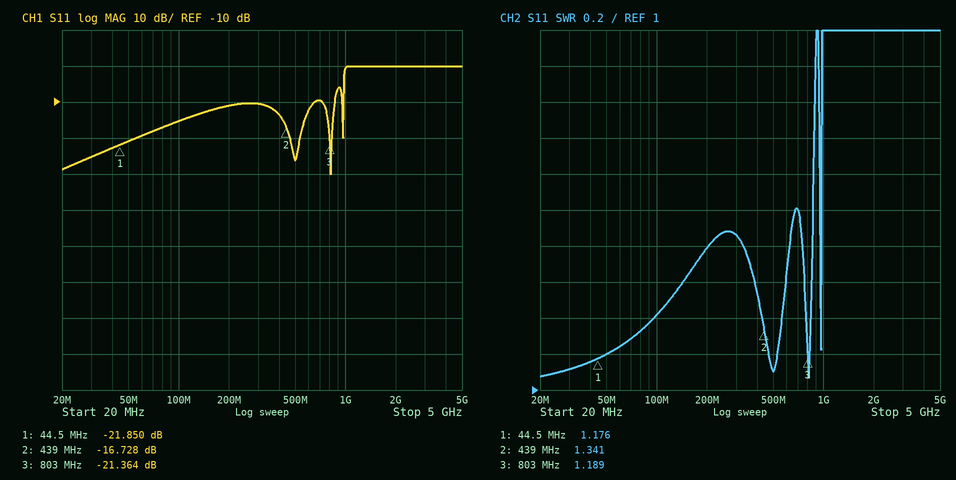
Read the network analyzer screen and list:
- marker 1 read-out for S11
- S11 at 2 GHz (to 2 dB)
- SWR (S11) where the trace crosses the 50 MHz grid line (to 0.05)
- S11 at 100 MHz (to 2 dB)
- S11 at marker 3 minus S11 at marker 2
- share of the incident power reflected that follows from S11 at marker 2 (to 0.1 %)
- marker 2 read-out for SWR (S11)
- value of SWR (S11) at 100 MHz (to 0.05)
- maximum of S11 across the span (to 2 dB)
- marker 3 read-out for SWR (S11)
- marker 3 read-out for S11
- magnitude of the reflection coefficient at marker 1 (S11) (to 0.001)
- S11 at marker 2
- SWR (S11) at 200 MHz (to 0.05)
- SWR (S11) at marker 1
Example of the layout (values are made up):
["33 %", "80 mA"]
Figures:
["-21.850 dB", "0 dB", "1.20", "-16 dB", "-4.636 dB", "2.1 %", "1.341", "1.40", "0 dB", "1.189", "-21.364 dB", "0.081", "-16.728 dB", "1.80", "1.176"]
